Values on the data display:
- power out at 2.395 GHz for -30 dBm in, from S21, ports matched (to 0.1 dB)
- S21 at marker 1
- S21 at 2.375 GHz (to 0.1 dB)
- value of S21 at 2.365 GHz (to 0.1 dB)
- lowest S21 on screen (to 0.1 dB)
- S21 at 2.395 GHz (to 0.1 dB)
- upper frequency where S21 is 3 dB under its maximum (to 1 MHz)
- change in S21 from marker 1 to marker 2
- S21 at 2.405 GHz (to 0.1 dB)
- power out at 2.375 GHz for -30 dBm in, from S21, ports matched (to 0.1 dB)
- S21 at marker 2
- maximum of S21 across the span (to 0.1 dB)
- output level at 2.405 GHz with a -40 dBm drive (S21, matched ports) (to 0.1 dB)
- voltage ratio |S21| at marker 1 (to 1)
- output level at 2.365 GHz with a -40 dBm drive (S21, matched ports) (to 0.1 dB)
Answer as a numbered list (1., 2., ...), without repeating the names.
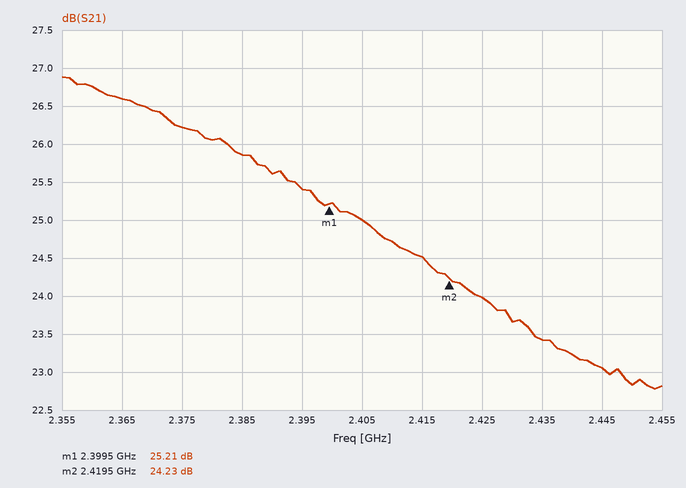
1. -4.6 dBm
2. 25.21 dB
3. 26.2 dB
4. 26.6 dB
5. 22.8 dB
6. 25.4 dB
7. 2.427 GHz
8. -0.98 dB
9. 25.0 dB
10. -3.8 dBm
11. 24.23 dB
12. 26.9 dB
13. -15.0 dBm
14. 18
15. -13.4 dBm
